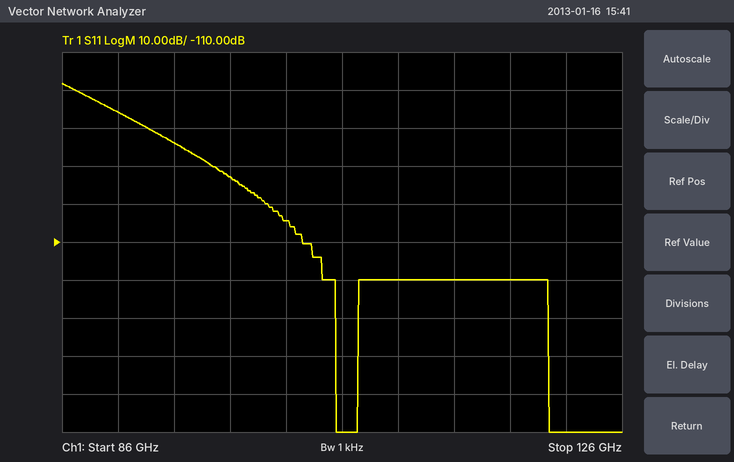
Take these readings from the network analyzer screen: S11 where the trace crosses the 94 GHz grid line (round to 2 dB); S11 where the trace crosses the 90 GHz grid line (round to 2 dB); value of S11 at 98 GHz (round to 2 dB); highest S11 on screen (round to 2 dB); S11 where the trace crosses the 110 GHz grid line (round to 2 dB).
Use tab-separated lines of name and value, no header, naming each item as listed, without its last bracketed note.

S11 where the trace crosses the 94 GHz grid line	-84 dB
S11 where the trace crosses the 90 GHz grid line	-76 dB
value of S11 at 98 GHz	-92 dB
highest S11 on screen	-68 dB
S11 where the trace crosses the 110 GHz grid line	-120 dB
